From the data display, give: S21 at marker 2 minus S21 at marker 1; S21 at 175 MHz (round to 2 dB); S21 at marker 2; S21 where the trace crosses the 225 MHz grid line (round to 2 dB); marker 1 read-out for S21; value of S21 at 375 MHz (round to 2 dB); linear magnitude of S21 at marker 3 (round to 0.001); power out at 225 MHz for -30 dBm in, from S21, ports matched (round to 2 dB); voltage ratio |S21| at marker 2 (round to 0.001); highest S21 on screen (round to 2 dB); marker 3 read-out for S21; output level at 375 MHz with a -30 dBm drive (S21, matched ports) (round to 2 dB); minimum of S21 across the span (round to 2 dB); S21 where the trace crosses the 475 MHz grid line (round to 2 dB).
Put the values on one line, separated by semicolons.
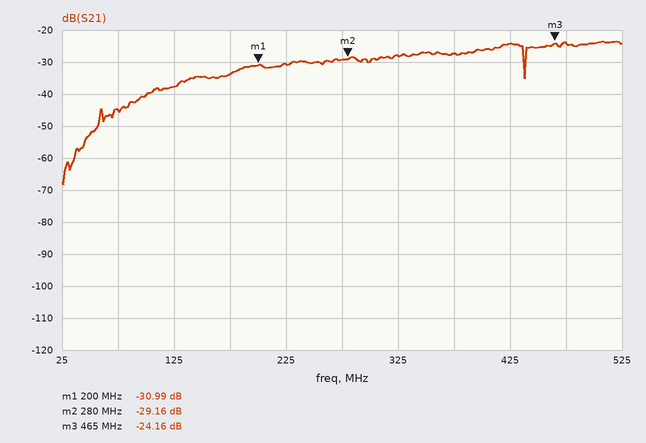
1.83 dB; -34 dB; -29.16 dB; -30 dB; -30.99 dB; -28 dB; 0.062; -60 dBm; 0.035; -24 dB; -24.16 dB; -58 dBm; -68 dB; -24 dB
